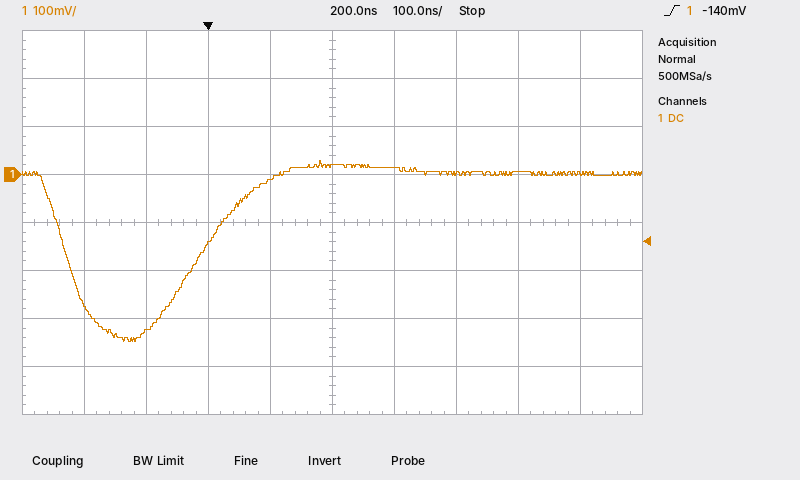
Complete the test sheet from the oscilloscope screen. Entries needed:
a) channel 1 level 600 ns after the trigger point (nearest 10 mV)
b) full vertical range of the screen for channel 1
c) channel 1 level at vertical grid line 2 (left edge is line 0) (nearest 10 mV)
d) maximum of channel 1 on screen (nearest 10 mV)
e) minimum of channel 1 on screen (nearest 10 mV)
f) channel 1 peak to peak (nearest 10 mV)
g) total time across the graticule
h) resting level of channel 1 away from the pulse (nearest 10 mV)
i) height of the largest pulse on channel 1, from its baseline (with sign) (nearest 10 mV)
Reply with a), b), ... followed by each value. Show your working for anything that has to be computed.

a) 0 mV
b) 800 mV
c) -330 mV
d) 30 mV
e) -350 mV
f) 30 mV − (-350 mV) = 380 mV
g) 1 µs
h) 0 mV
i) -350 mV − (0 mV) = -350 mV
